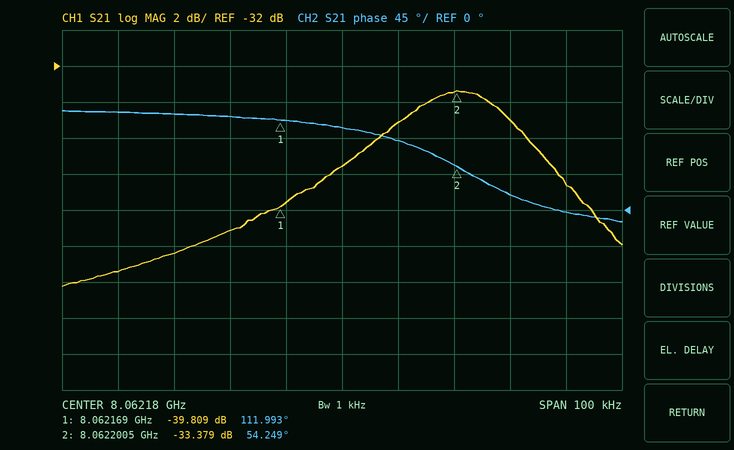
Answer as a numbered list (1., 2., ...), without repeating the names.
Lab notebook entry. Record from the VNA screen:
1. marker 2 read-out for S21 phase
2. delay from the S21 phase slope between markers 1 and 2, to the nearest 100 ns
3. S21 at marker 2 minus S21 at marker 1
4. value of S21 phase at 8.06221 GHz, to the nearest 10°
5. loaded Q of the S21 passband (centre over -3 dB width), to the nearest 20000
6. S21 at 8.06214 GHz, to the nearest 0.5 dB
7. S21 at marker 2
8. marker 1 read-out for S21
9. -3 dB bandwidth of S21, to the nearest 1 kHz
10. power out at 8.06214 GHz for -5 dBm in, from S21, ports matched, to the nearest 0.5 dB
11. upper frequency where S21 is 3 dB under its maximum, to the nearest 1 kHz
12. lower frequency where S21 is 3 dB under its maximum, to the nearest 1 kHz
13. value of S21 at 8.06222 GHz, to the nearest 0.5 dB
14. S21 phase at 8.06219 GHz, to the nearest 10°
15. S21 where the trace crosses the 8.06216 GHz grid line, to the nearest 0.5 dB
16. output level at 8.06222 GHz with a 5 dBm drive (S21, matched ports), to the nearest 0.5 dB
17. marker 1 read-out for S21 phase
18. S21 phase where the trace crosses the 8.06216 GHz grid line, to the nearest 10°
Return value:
1. 54.249°
2. 5.1 µs
3. 6.430 dB
4. 20°
5. 280000
6. -43.5 dB
7. -33.379 dB
8. -39.809 dB
9. 29 kHz
10. -48.5 dBm
11. 8.062214 GHz
12. 8.062185 GHz
13. -38.5 dB
14. 90°
15. -41.0 dB
16. -33.5 dBm
17. 111.993°
18. 120°
